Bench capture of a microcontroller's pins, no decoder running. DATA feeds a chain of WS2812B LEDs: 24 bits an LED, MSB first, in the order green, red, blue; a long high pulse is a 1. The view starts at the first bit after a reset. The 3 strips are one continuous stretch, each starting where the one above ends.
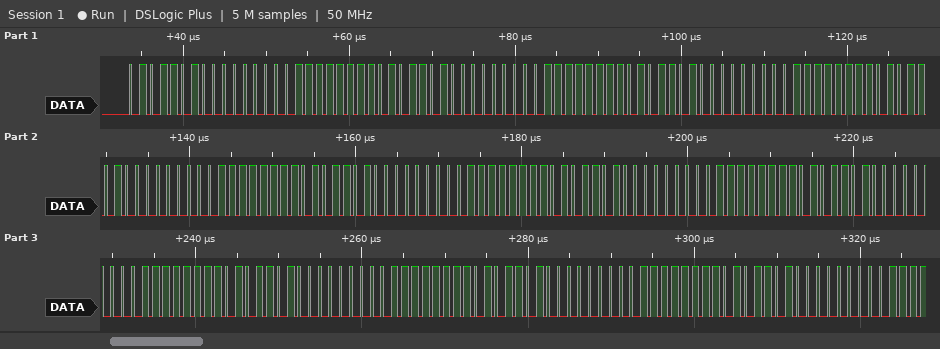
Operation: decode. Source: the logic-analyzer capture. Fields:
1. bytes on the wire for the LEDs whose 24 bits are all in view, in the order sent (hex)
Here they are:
5A 00 FF 5A 00 FF 5A 00 FF 5A 00 FF 5A 00 FF 5A 00 FF 5A 00 FF 5A 00 FF 5A 00 FF
